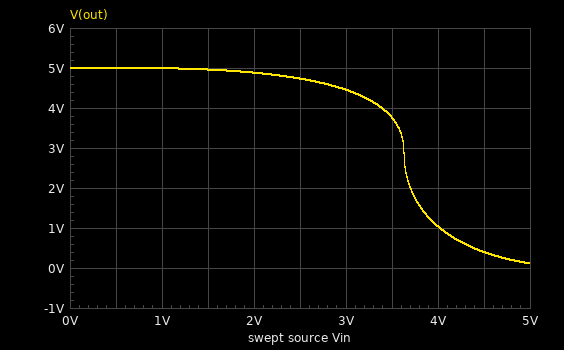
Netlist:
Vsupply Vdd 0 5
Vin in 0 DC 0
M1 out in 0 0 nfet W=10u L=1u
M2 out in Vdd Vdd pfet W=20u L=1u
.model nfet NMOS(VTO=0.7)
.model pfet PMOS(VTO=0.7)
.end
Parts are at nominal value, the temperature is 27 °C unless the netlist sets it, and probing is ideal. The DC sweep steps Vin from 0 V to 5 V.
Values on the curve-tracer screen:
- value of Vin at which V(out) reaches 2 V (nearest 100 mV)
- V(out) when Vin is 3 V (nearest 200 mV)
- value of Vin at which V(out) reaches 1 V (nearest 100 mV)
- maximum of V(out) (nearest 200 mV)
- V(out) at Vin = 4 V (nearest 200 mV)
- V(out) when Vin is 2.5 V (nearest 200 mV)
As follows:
3.7 V
4.4 V
4.0 V
5.0 V
1.0 V
4.8 V
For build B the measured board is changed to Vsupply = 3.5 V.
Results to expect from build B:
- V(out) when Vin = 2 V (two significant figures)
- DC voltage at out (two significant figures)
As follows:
3.3 V
3.5 V
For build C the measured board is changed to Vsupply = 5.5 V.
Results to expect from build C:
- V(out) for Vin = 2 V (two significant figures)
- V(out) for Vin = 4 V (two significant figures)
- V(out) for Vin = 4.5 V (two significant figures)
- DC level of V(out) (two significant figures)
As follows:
5.4 V
2.2 V
860 mV
5.5 V
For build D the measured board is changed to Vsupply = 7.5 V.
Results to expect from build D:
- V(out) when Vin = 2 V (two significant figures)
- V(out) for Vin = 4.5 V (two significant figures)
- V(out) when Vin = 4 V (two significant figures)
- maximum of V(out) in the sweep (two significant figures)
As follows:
7.4 V
6.3 V
6.8 V
7.5 V
